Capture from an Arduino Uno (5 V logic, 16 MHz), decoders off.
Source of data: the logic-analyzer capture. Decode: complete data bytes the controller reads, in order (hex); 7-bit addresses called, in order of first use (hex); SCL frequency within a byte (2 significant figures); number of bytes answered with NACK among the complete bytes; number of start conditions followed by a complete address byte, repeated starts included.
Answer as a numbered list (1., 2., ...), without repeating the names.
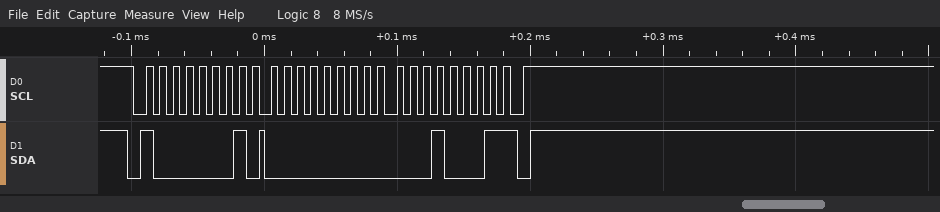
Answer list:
1. 00 11
2. 0x40
3. 100 kHz
4. 1
5. 1
